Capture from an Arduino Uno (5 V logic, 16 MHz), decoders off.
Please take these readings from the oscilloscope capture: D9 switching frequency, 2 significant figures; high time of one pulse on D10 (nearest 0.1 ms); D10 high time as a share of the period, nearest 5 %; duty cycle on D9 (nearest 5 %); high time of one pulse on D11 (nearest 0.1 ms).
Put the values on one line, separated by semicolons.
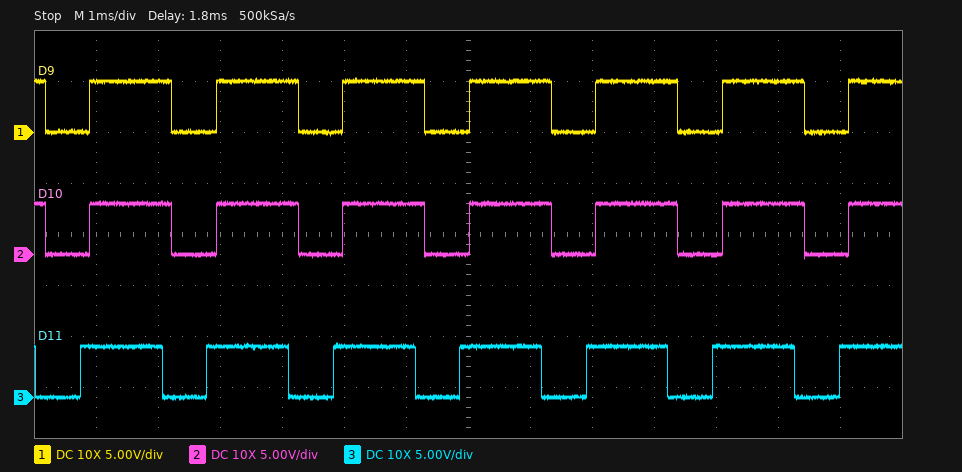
490 Hz; 1.3 ms; 65 %; 65 %; 1.3 ms
